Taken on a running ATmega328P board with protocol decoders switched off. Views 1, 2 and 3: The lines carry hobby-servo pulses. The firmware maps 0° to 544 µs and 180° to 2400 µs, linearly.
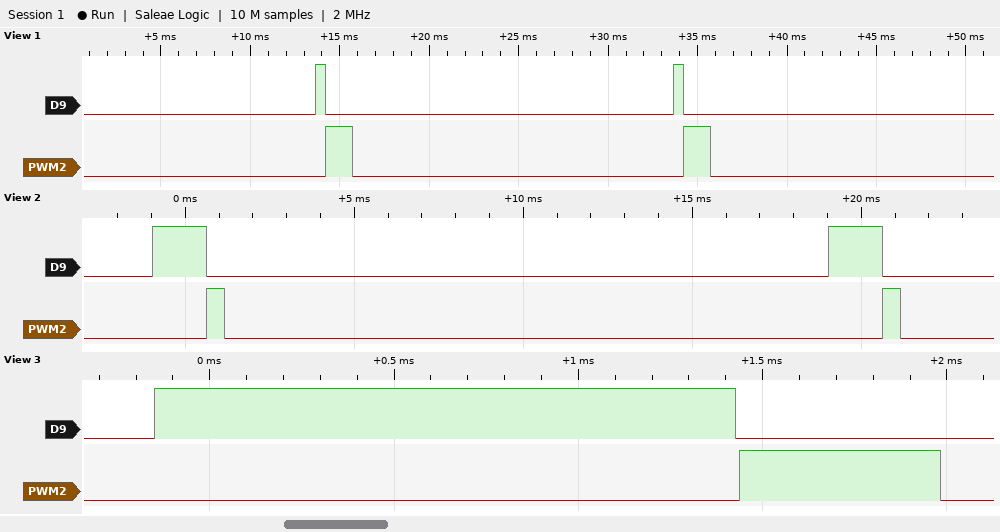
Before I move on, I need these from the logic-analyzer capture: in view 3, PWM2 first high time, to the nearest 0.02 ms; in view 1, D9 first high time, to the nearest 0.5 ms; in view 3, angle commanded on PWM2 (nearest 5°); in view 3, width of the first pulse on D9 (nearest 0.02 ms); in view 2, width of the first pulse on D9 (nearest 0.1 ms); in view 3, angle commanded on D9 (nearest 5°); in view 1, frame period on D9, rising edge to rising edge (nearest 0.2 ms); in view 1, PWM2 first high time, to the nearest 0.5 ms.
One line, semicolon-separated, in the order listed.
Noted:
0.54 ms; 0.5 ms; 0°; 1.58 ms; 1.6 ms; 100°; 20.0 ms; 1.5 ms
